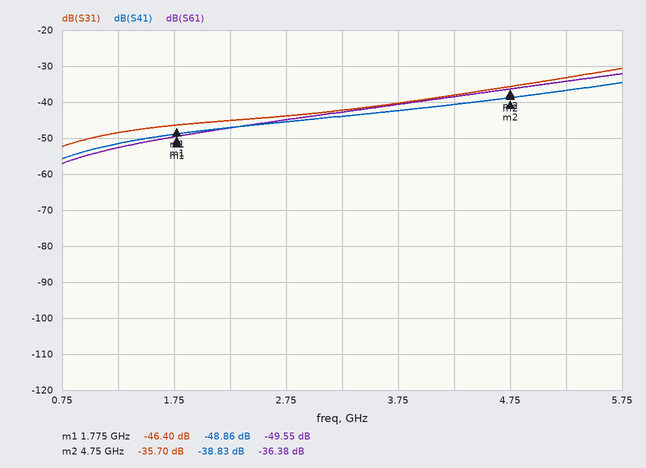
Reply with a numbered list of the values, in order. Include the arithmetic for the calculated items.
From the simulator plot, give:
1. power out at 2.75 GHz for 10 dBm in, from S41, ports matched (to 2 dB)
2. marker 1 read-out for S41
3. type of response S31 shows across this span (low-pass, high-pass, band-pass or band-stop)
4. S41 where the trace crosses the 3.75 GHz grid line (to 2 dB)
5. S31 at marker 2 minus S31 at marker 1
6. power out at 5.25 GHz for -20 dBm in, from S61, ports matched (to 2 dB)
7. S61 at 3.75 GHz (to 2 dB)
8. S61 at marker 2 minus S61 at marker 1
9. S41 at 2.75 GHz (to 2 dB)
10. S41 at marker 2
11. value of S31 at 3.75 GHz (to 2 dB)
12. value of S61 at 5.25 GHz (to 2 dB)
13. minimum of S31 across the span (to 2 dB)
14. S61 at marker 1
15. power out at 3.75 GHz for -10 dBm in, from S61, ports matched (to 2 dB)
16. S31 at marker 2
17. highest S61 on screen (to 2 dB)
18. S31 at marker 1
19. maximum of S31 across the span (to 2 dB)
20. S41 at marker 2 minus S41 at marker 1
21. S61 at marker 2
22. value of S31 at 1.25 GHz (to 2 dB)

1. 10 dBm + (-46 dB) = -36 dBm
2. -48.86 dB
3. high-pass
4. -42 dB
5. -35.7 − (-46.4) = 10.70 dB
6. -20 dBm + (-34 dB) = -54 dBm
7. -40 dB
8. -36.38 − (-49.55) = 13.17 dB
9. -46 dB
10. -38.83 dB
11. -40 dB
12. -34 dB
13. -52 dB
14. -49.55 dB
15. -10 dBm + (-40 dB) = -50 dBm
16. -35.70 dB
17. -32 dB
18. -46.40 dB
19. -30 dB
20. -38.83 − (-48.86) = 10.03 dB
21. -36.38 dB
22. -48 dB
